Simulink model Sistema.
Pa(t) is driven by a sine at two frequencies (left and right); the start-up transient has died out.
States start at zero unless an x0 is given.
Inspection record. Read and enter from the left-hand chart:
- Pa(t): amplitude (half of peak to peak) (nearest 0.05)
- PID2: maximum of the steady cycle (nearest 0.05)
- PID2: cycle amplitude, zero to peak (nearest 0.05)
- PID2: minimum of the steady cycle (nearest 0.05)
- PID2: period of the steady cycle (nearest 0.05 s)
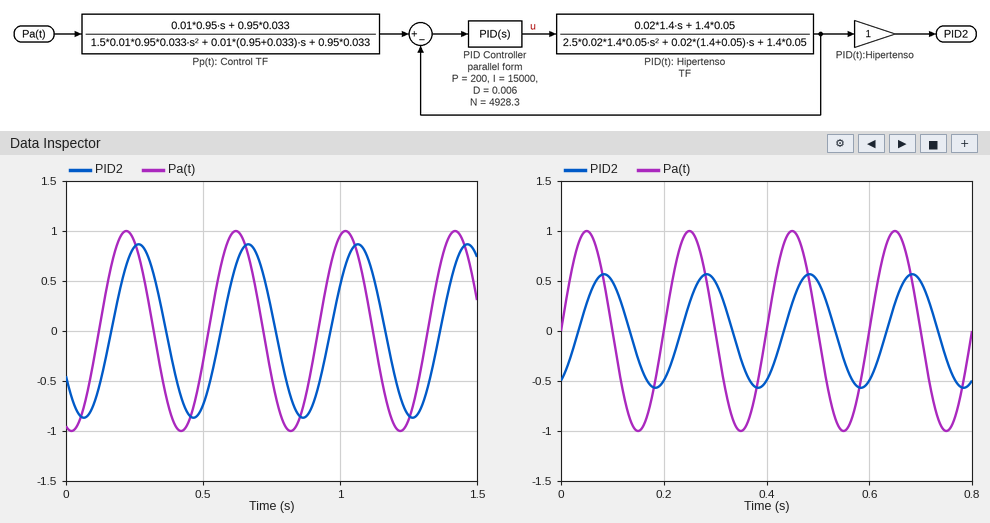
1.00
0.85
0.85
-0.85
0.40 s
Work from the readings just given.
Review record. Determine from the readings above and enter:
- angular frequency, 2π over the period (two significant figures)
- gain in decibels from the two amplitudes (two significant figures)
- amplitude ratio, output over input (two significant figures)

16 rad/s
-1.4 dB
0.85
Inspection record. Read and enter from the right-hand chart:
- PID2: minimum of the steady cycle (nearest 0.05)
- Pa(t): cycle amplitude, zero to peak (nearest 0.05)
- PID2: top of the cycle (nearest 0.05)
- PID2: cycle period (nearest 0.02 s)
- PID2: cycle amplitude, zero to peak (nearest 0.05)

-0.55
1.00
0.55
0.20 s
0.55
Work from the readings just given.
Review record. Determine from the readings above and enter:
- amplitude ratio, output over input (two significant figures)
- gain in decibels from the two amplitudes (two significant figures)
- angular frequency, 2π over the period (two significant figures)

0.55
-5.2 dB
31 rad/s
